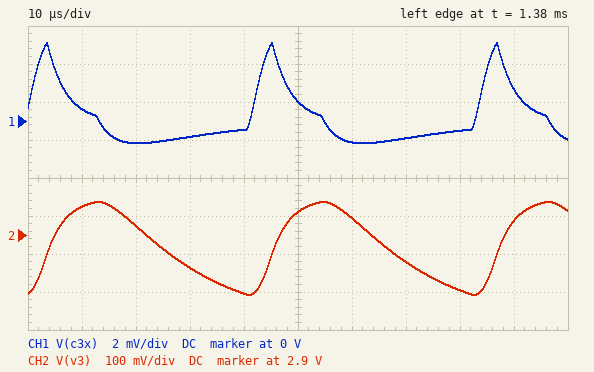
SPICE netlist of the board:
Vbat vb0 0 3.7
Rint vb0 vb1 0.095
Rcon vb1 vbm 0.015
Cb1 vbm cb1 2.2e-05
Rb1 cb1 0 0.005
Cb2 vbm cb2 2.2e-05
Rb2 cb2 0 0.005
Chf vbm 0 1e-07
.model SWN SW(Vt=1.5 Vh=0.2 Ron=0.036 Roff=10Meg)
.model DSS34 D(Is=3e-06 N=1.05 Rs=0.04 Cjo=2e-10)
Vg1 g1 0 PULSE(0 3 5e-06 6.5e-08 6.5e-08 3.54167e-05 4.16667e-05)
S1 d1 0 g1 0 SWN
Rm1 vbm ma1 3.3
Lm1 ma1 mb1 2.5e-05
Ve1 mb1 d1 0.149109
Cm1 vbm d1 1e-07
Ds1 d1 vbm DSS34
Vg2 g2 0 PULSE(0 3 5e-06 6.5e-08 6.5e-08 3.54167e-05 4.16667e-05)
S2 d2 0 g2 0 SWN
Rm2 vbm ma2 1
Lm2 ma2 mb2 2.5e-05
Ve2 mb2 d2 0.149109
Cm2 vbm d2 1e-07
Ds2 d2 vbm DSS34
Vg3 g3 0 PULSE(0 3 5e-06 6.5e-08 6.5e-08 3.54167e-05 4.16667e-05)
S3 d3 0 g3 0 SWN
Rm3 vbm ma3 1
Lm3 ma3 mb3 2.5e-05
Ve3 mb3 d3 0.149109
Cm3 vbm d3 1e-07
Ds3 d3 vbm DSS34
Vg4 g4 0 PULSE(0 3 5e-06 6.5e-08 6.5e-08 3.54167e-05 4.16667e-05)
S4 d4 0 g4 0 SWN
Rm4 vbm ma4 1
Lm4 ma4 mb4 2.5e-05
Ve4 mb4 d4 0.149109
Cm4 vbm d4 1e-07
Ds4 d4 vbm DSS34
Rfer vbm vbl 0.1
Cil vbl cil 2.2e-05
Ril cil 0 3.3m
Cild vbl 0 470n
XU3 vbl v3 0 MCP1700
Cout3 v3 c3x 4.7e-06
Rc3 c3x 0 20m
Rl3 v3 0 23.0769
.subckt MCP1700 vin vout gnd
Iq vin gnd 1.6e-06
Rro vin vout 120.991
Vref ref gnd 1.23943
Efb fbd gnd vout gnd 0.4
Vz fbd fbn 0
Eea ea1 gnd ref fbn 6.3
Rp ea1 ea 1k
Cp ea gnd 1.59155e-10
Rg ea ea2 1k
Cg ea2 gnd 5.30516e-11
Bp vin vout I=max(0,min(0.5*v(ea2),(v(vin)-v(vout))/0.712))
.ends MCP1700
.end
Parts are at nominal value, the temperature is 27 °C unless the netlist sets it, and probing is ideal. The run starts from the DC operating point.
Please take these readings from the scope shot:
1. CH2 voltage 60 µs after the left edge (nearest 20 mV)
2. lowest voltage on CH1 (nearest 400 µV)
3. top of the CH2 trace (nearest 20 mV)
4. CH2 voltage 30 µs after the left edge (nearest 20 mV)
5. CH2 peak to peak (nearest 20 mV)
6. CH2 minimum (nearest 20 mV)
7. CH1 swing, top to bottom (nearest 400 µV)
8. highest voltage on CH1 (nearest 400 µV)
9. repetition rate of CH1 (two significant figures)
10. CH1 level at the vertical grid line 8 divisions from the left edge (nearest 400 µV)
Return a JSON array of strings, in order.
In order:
["2.94 V", "-1.2 mV", "2.98 V", "2.82 V", "240 mV", "2.74 V", "5.2 mV", "4.0 mV", "24 kHz", "-400 µV"]
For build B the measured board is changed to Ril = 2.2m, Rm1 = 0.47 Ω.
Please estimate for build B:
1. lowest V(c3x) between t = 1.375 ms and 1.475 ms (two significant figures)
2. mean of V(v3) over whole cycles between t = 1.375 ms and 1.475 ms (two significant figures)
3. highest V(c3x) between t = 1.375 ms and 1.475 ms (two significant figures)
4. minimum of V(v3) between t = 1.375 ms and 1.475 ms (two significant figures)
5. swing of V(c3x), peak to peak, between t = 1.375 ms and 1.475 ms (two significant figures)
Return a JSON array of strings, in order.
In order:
["-1.8 mV", "2.6 V", "6.1 mV", "2.5 V", "7.9 mV"]
